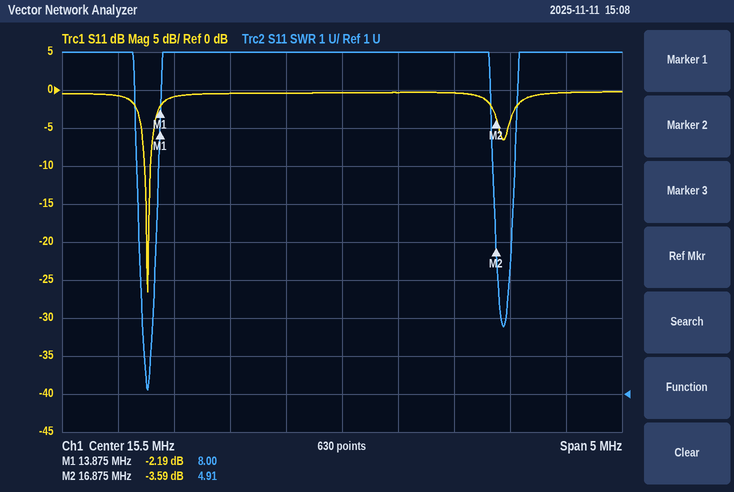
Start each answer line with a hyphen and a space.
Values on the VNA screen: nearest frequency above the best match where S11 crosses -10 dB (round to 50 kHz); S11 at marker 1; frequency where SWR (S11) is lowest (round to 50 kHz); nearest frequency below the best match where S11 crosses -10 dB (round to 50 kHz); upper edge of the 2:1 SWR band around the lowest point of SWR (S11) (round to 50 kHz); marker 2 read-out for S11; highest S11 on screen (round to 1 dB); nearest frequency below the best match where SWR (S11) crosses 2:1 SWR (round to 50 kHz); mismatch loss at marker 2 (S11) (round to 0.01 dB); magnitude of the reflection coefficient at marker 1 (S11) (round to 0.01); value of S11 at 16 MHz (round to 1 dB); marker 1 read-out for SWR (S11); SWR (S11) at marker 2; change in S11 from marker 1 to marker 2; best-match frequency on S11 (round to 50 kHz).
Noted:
- 13.80 MHz
- -2.19 dB
- 13.75 MHz
- 13.75 MHz
- 13.80 MHz
- -3.59 dB
- 0 dB
- 13.75 MHz
- 2.50 dB
- 0.78
- 0 dB
- 8.00
- 4.91
- -1.40 dB
- 13.75 MHz
